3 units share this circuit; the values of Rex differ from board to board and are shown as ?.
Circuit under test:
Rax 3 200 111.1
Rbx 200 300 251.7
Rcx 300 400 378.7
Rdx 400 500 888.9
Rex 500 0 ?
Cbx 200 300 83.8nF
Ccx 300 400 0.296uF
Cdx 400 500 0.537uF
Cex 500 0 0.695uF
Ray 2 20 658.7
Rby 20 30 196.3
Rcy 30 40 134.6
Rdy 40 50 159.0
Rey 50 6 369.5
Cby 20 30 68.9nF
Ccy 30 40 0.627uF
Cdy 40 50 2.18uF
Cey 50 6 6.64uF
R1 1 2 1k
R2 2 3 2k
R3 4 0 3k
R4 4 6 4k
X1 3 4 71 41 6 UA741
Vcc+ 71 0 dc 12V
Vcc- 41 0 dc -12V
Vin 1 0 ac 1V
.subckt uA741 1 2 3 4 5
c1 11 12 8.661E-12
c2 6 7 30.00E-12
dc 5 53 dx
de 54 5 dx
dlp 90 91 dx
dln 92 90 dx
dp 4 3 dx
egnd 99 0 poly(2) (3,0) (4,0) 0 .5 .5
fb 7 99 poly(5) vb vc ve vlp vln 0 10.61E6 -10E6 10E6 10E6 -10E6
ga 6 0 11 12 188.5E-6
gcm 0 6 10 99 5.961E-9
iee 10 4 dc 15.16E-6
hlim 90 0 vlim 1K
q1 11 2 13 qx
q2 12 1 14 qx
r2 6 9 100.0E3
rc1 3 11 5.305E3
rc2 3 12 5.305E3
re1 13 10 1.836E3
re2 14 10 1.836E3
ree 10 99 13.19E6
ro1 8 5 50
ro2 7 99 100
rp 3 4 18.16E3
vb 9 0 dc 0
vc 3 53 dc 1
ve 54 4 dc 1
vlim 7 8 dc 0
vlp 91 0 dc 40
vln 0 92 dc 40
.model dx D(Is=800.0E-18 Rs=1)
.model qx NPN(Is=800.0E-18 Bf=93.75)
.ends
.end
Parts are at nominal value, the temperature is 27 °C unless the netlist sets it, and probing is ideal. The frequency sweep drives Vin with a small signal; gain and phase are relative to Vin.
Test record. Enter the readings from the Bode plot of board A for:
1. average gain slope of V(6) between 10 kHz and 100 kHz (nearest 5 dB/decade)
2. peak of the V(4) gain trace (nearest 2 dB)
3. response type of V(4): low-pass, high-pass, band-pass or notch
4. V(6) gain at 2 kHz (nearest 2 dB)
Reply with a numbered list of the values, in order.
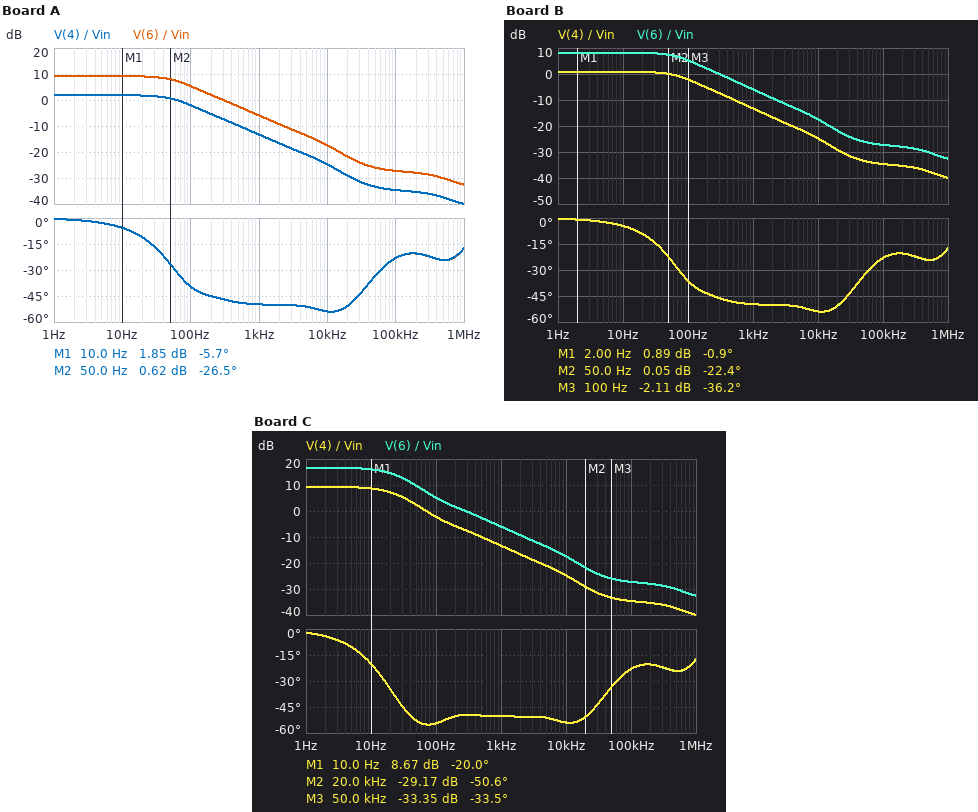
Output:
1. -10 dB/decade
2. 2 dB
3. low-pass
4. -10 dB
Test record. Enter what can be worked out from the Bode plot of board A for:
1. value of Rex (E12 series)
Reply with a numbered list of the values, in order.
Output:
1. 4.7 kΩ
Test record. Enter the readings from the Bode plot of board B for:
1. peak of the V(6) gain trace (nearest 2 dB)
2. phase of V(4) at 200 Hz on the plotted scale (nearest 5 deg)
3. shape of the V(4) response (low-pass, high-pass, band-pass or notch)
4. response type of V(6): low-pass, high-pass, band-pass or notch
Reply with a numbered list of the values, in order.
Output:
1. 8 dB
2. -45 deg
3. low-pass
4. low-pass
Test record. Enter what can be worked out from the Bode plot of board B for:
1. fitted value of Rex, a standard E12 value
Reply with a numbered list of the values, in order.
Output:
1. 3.9 kΩ
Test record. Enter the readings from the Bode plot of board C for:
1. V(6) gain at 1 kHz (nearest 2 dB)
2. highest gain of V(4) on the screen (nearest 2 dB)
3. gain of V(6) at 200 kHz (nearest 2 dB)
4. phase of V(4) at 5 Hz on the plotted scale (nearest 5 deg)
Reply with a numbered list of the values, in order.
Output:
1. -6 dB
2. 10 dB
3. -28 dB
4. -10 deg
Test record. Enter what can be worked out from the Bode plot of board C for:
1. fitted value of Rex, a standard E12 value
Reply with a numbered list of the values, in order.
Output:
1. 18 kΩ
